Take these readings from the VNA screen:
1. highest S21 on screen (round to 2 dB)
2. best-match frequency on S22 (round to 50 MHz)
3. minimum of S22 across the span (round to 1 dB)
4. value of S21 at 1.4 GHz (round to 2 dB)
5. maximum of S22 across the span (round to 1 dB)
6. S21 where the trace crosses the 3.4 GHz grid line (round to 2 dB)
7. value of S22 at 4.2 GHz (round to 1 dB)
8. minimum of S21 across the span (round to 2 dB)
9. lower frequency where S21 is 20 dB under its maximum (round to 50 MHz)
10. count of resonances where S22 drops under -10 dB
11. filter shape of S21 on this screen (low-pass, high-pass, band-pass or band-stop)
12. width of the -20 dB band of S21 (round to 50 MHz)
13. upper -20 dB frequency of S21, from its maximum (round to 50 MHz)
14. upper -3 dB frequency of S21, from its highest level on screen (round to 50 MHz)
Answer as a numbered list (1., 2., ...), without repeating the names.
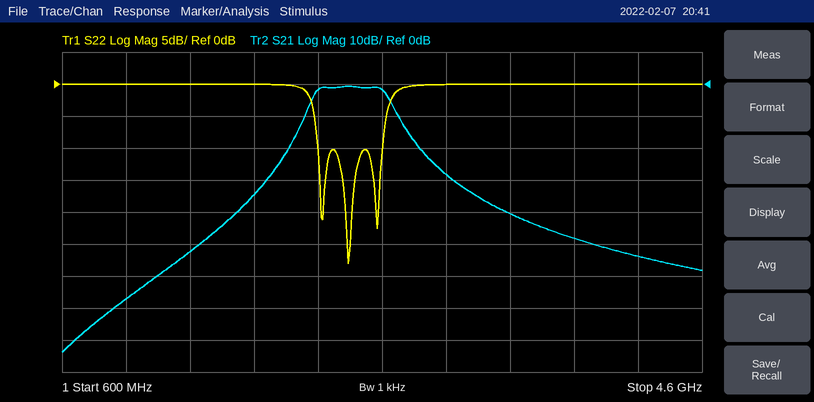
1. 0 dB
2. 2.40 GHz
3. -28 dB
4. -52 dB
5. 0 dB
6. -40 dB
7. 0 dB
8. -84 dB
9. 2.00 GHz
10. 3
11. band-pass
12. 850 MHz
13. 2.85 GHz
14. 2.65 GHz
